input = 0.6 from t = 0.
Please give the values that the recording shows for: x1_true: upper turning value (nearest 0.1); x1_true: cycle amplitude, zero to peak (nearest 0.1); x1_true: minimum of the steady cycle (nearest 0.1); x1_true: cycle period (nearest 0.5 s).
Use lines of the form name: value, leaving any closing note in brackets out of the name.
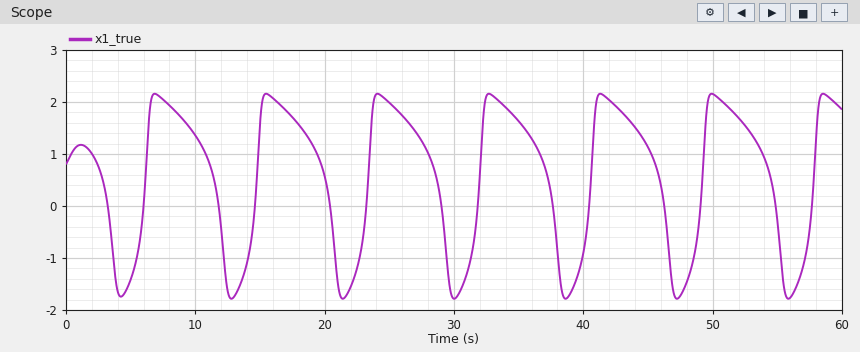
x1_true: upper turning value: 2.2
x1_true: cycle amplitude, zero to peak: 2.0
x1_true: minimum of the steady cycle: -1.8
x1_true: cycle period: 8.5 s
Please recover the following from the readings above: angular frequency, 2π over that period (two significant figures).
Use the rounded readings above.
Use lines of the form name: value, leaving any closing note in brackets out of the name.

angular frequency, 2π over that period: 0.74 rad/s
